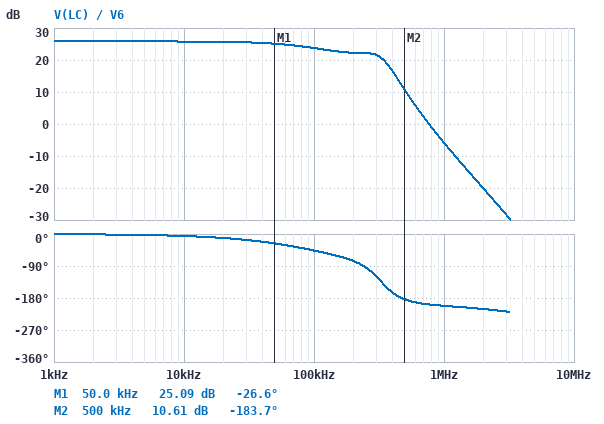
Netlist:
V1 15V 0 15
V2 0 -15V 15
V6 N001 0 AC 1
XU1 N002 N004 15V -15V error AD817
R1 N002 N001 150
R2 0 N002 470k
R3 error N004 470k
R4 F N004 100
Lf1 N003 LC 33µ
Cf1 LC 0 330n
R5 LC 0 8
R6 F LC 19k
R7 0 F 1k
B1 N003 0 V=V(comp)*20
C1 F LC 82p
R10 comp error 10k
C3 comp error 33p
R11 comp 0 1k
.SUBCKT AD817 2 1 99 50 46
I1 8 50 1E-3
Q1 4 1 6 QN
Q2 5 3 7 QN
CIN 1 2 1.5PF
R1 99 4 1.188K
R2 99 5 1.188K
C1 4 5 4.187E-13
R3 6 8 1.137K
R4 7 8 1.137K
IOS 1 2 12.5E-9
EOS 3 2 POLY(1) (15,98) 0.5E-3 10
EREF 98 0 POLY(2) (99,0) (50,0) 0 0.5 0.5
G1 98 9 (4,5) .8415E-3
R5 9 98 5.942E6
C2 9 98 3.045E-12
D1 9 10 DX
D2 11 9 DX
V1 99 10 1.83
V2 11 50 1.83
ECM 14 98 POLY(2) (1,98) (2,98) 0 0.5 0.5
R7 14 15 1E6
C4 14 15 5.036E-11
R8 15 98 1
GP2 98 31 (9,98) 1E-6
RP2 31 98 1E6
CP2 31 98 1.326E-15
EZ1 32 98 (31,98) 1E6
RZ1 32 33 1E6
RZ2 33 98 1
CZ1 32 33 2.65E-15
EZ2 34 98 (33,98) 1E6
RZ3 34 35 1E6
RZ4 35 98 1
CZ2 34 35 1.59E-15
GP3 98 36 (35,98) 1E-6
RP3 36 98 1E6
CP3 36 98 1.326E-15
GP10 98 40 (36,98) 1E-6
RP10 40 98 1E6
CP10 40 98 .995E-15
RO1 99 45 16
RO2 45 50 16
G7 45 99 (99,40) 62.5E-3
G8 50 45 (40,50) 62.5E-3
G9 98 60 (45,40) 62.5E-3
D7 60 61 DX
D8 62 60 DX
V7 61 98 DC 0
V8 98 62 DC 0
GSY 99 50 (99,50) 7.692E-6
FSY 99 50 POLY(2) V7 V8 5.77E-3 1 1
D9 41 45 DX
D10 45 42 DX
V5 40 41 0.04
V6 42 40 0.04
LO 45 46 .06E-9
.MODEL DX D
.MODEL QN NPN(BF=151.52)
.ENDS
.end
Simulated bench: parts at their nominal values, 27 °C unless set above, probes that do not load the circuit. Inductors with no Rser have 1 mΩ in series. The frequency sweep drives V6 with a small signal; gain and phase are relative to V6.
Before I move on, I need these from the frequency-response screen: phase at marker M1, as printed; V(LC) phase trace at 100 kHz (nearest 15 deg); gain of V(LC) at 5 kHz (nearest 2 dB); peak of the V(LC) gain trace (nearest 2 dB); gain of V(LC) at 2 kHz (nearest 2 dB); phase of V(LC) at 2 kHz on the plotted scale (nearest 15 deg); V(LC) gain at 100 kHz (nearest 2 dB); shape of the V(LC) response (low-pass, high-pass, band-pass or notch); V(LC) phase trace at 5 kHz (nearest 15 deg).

-26.6 deg
-45 deg
26 dB
26 dB
26 dB
0 deg
24 dB
low-pass
0 deg
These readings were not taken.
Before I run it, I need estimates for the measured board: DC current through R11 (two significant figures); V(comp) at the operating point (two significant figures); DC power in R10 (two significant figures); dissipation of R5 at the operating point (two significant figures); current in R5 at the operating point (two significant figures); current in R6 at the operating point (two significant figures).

3.4 µA
3.4 mV
110 nW
570 µW
8.4 mA
3.5 µA
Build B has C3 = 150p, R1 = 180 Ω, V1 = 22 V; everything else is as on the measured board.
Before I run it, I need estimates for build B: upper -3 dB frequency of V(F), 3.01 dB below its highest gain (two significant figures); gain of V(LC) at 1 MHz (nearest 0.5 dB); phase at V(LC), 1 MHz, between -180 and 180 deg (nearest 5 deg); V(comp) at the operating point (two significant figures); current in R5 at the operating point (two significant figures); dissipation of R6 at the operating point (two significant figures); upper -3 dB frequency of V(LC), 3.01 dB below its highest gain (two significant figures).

1.0 MHz
9.0 dB
165 deg
3.9 mV
9.8 mA
320 nW
110 kHz
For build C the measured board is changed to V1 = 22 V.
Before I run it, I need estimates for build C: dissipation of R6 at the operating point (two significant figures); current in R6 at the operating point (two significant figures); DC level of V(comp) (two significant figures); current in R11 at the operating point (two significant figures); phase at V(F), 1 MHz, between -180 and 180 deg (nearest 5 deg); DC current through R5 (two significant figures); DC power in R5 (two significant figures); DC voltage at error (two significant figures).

330 nW
4.2 µA
4.0 mV
4.0 µA
-135 deg
10 mA
810 µW
44 mV
